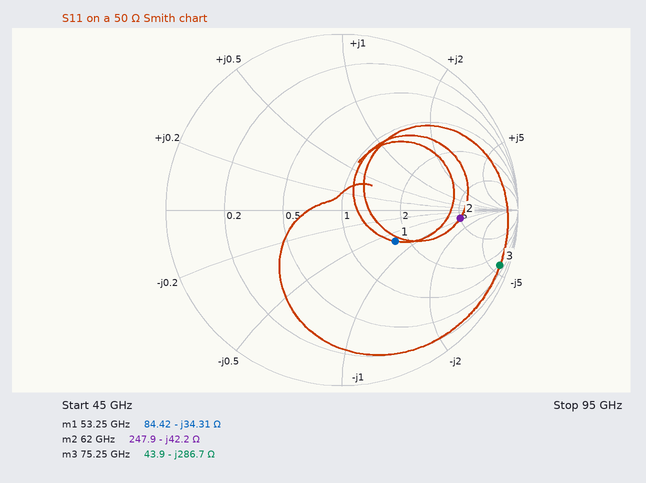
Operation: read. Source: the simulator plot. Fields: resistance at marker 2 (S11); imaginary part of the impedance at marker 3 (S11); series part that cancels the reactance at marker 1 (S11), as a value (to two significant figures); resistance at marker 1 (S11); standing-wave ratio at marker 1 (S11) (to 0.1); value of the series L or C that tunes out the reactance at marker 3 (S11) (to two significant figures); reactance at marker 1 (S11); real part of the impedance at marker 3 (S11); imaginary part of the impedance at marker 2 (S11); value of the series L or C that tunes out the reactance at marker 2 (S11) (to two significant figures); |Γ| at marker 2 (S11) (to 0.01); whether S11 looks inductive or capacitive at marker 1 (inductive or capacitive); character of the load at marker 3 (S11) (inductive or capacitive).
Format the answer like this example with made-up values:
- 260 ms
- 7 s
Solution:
- 247.9 Ω
- -286.7 Ω
- 100 pH
- 84.42 Ω
- 2.1
- 610 pH
- -34.31 Ω
- 43.9 Ω
- -42.2 Ω
- 110 pH
- 0.67
- capacitive
- capacitive
